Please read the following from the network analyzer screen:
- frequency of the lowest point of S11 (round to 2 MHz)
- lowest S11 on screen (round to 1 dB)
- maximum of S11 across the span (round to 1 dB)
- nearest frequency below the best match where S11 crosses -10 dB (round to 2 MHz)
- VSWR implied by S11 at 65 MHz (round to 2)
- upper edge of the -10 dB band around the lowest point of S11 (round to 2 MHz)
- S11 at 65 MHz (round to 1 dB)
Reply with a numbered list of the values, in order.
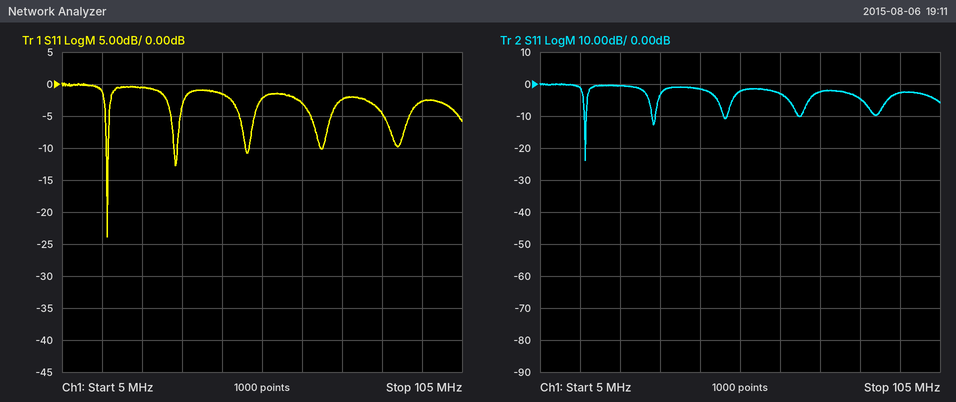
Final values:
1. 16 MHz
2. -24 dB
3. 0 dB
4. 16 MHz
5. 6
6. 16 MHz
7. -3 dB
